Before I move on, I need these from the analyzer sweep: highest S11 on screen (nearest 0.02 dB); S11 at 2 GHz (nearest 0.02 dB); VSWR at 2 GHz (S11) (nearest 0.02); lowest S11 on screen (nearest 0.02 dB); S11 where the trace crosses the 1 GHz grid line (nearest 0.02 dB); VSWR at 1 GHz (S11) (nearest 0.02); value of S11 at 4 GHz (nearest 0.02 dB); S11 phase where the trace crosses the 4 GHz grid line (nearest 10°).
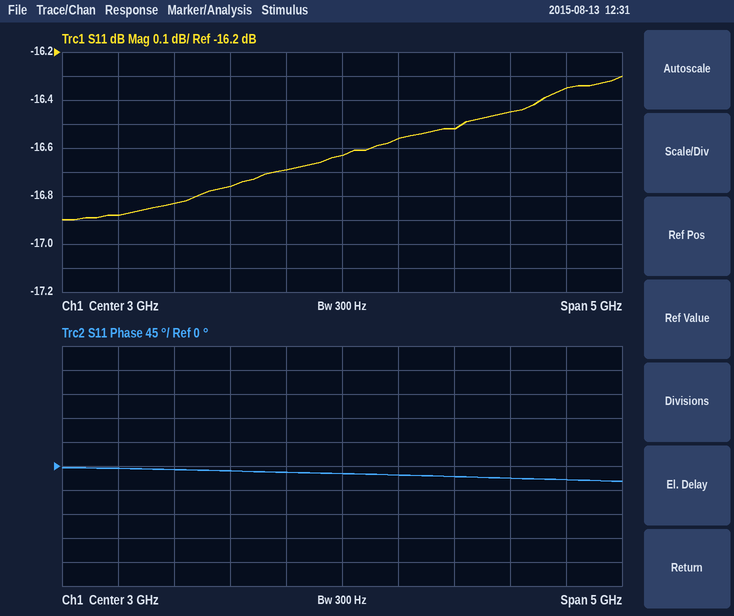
-16.30 dB
-16.76 dB
1.34
-16.90 dB
-16.88 dB
1.34
-16.52 dB
-20°
